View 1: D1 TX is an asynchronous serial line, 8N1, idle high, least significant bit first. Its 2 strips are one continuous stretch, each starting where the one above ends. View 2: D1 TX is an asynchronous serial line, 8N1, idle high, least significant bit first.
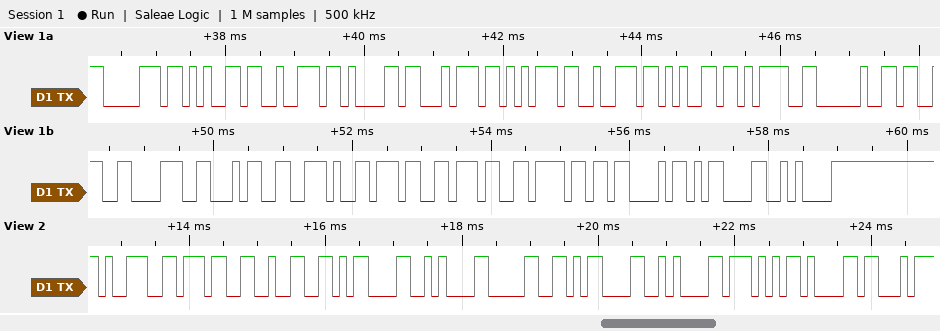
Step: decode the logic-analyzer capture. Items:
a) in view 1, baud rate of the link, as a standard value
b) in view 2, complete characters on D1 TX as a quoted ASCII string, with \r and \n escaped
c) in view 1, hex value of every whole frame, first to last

9600 baud
"972\r\n0\r\nWa"
70 65 72 61 74 75 72 65 3D 20 33 38 34 2E 37 37 6F 43 0D 0A
